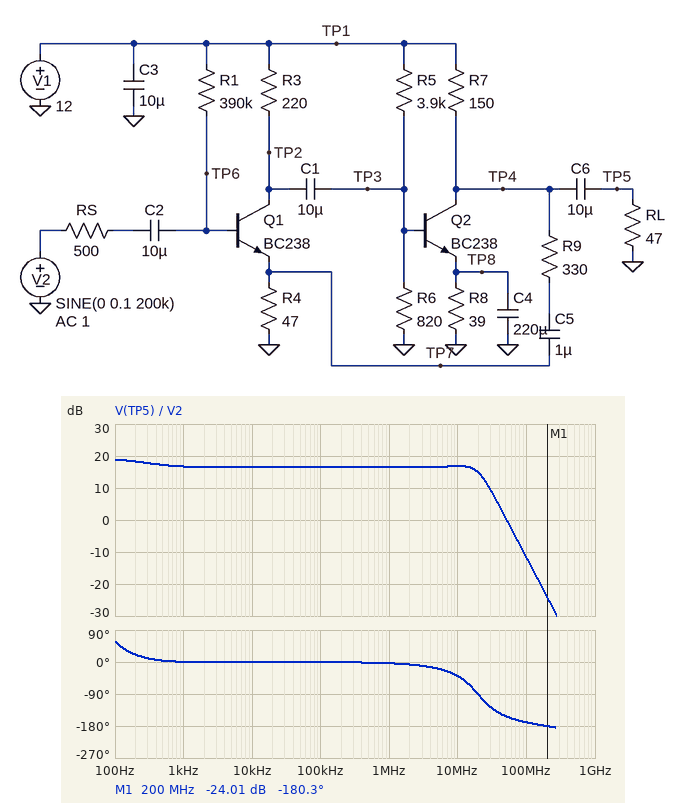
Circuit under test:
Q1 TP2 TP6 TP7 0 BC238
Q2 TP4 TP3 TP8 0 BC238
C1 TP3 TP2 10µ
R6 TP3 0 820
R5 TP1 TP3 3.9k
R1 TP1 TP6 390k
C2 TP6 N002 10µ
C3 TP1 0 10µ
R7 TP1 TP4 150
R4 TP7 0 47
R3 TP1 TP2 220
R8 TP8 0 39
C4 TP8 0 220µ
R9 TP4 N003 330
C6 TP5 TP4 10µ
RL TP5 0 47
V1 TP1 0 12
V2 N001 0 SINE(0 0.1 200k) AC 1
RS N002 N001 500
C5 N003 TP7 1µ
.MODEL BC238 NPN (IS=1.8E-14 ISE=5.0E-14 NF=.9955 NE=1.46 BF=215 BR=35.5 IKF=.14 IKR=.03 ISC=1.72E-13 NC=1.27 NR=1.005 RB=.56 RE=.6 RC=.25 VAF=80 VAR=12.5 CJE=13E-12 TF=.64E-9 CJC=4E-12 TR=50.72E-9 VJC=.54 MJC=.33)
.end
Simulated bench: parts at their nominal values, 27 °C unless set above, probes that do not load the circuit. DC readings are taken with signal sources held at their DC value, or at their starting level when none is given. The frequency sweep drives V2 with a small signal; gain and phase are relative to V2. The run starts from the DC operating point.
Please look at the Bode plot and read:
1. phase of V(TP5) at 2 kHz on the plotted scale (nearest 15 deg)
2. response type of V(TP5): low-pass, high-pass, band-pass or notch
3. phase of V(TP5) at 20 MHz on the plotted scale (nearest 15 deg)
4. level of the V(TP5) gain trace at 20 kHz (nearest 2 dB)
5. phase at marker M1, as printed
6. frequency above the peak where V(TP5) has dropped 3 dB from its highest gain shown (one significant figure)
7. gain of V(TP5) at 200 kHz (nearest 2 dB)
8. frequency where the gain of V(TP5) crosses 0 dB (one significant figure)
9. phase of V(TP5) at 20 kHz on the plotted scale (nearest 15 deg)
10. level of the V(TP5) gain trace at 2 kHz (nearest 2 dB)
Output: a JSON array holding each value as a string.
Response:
["0 deg", "low-pass", "-90 deg", "16 dB", "-180.3 deg", "20 MHz", "16 dB", "50 MHz", "0 deg", "16 dB"]
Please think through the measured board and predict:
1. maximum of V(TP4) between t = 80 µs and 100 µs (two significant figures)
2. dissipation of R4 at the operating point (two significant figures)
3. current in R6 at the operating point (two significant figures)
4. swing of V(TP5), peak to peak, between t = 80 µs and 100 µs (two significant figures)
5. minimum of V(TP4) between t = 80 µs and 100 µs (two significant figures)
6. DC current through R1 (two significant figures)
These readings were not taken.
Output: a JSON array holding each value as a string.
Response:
["8.0 V", "1.5 mW", "2.4 mA", "1.3 V", "6.7 V", "28 µA"]
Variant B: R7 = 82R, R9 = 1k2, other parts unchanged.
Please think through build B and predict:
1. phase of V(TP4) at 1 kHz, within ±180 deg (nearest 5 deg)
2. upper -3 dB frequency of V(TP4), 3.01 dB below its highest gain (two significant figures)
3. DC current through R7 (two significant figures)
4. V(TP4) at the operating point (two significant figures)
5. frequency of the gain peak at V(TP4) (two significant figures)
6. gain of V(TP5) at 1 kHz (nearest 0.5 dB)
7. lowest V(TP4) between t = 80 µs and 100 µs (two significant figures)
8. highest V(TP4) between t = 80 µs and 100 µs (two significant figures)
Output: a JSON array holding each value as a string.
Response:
["0 deg", "530 Hz", "31 mA", "9.5 V", "95 Hz", "23.0 dB", "8.0 V", "10 V"]
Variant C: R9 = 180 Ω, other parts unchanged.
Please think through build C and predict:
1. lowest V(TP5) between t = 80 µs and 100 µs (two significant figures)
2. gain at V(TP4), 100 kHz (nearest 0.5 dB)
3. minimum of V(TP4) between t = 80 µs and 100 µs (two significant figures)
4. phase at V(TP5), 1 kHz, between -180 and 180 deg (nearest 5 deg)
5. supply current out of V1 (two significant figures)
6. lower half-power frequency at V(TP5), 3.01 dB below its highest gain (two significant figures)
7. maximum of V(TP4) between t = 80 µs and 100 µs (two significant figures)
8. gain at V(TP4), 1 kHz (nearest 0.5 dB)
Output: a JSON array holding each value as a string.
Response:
["-430 mV", "12.5 dB", "6.9 V", "-10 deg", "39 mA", "64 Hz", "7.8 V", "14.5 dB"]
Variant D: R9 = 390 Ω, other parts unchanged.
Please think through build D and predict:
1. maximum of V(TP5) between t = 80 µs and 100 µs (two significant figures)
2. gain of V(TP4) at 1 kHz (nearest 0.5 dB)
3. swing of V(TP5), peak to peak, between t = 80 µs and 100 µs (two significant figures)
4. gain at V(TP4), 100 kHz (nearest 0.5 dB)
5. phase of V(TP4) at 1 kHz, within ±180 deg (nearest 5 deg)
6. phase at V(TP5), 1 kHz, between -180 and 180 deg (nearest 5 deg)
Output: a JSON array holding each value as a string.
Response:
["730 mV", "18.0 dB", "1.5 V", "17.5 dB", "-15 deg", "5 deg"]
